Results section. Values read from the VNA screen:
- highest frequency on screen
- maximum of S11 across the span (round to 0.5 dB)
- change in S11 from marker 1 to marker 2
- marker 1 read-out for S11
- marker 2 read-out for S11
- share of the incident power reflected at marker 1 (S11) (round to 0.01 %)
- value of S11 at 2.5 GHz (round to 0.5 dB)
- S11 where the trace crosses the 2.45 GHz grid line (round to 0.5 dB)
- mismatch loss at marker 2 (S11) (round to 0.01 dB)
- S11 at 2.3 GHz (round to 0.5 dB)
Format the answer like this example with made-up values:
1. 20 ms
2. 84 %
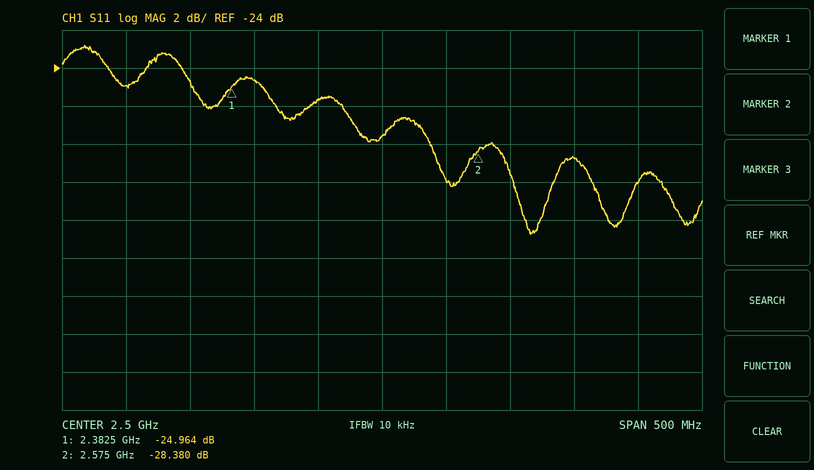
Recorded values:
1. 2.75 GHz
2. -23.0 dB
3. -3.416 dB
4. -24.964 dB
5. -28.380 dB
6. 0.32 %
7. -27.5 dB
8. -25.5 dB
9. 0.01 dB
10. -25.0 dB
